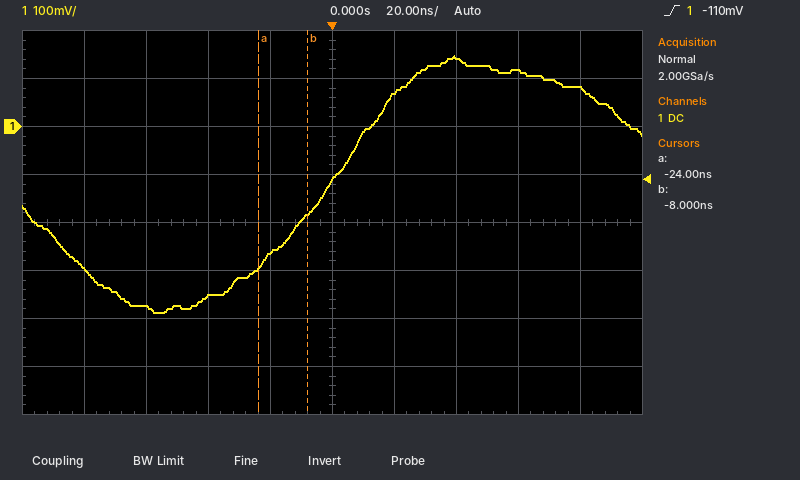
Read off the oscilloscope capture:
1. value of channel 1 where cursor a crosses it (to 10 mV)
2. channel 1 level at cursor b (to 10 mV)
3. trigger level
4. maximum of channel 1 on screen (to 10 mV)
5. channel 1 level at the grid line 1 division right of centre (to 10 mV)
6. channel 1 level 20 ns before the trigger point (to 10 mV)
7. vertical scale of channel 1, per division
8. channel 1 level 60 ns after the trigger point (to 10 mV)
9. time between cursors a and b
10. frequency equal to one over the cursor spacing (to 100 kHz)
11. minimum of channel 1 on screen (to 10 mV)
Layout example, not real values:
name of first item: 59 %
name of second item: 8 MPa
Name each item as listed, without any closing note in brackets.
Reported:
value of channel 1 where cursor a crosses it: -290 mV
channel 1 level at cursor b: -180 mV
trigger level: -110 mV
maximum of channel 1 on screen: 150 mV
channel 1 level at the grid line 1 division right of centre: 70 mV
channel 1 level 20 ns before the trigger point: -260 mV
vertical scale of channel 1, per division: 100 mV
channel 1 level 60 ns after the trigger point: 120 mV
time between cursors a and b: 16 ns
frequency equal to one over the cursor spacing: 62.5 MHz
minimum of channel 1 on screen: -390 mV
